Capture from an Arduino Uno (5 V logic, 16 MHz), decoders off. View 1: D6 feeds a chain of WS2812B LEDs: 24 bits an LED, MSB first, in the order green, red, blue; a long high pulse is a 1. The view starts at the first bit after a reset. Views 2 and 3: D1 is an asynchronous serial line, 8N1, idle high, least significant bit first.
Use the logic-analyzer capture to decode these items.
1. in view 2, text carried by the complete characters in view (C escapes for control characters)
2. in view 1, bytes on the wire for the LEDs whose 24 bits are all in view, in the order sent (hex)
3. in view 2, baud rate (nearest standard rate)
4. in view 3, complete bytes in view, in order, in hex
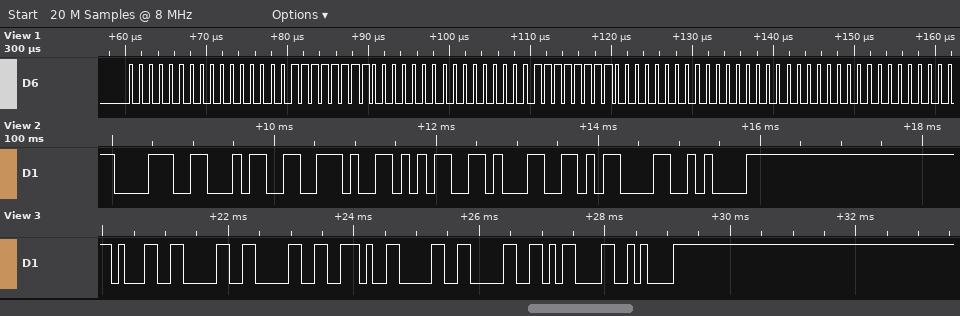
"84.51\r\n"
00 00 FF 00 00 FF 00 00 00
9600 baud
31 30 30 2E 30 30 0D 0A
